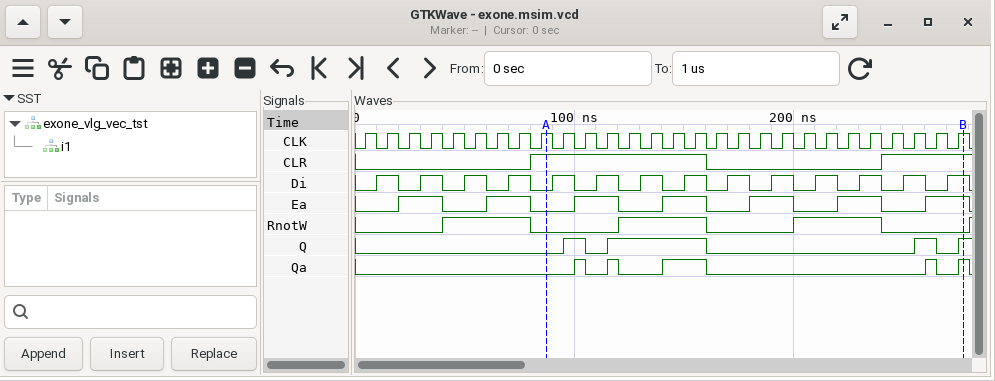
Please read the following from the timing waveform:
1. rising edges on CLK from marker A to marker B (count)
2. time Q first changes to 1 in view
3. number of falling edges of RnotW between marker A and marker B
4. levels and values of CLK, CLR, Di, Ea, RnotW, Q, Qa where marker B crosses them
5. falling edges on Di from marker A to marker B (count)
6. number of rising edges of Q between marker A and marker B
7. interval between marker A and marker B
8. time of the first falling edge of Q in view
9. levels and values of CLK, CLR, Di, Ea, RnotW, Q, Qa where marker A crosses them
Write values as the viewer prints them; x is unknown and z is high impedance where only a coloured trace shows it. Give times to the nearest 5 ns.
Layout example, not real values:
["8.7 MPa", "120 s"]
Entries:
["19", "95 ns", "2", "CLK=1, CLR=1, Di=1, Ea=1, RnotW=0, Q=1, Qa=1", "9", "4", "190 ns", "105 ns", "CLK=1, CLR=1, Di=0, Ea=0, RnotW=0, Q=0, Qa=0"]
